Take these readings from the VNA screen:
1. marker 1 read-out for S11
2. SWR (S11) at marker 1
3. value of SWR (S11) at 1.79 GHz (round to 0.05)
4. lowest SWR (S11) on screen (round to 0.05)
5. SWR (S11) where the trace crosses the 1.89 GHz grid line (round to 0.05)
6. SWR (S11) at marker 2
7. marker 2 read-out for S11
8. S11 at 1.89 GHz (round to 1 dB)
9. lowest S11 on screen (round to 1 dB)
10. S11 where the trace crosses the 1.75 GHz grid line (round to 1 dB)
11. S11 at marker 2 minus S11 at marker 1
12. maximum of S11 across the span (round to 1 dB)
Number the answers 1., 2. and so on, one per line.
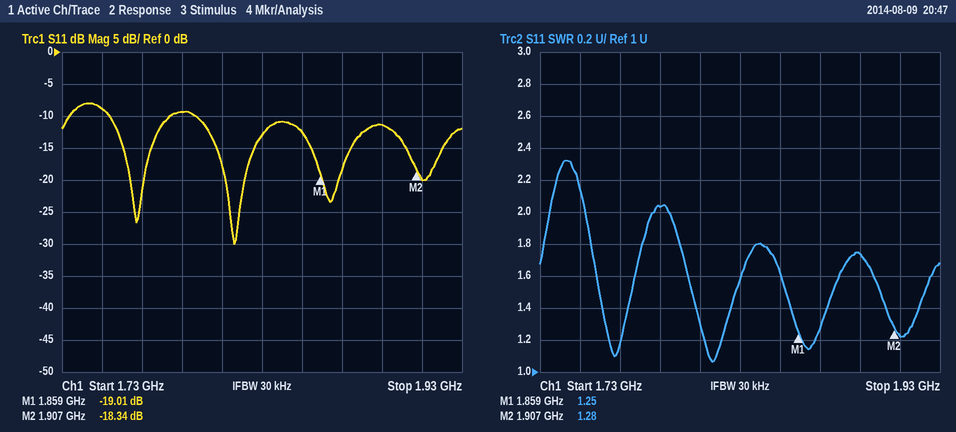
1. -19.01 dB
2. 1.25
3. 2.05
4. 1.05
5. 1.75
6. 1.28
7. -18.34 dB
8. -11 dB
9. -30 dB
10. -9 dB
11. 0.67 dB
12. -8 dB
